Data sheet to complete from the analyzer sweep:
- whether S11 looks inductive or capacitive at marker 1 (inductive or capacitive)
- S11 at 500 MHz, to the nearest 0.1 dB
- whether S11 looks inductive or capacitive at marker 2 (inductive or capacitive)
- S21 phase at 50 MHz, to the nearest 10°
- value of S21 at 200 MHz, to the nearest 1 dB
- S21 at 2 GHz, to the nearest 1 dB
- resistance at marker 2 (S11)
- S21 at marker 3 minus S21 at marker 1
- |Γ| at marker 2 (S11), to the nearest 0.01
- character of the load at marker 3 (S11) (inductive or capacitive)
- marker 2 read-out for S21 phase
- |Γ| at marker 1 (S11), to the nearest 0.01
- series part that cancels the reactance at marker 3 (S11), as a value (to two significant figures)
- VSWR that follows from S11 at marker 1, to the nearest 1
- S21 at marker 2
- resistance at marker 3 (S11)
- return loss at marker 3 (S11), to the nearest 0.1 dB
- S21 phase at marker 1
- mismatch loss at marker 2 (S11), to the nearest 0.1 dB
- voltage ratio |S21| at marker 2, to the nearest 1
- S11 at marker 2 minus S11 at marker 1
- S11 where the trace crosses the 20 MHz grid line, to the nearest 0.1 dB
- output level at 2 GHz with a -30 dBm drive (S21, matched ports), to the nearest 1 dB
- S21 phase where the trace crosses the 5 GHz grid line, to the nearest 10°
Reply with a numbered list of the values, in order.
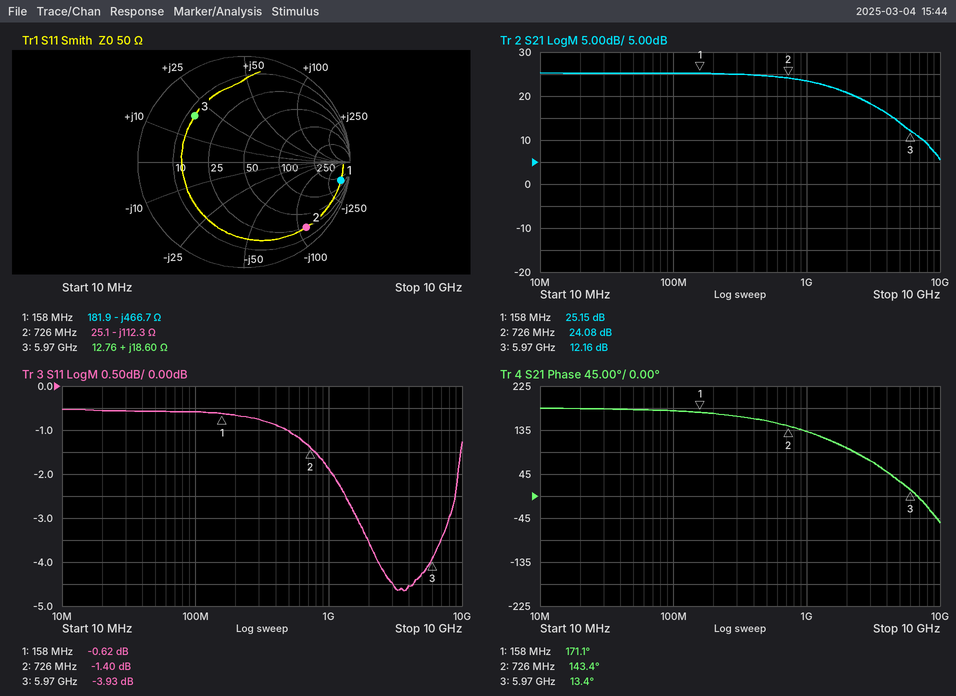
1. capacitive
2. -1.0 dB
3. capacitive
4. 180°
5. 25 dB
6. 21 dB
7. 25.1 Ω
8. -12.99 dB
9. 0.85
10. inductive
11. 143.4°
12. 0.93
13. 1.4 pF
14. 28
15. 24.08 dB
16. 12.76 Ω
17. 3.9 dB
18. 171.1°
19. 5.6 dB
20. 16
21. -0.78 dB
22. -0.6 dB
23. -9 dBm
24. 30°
